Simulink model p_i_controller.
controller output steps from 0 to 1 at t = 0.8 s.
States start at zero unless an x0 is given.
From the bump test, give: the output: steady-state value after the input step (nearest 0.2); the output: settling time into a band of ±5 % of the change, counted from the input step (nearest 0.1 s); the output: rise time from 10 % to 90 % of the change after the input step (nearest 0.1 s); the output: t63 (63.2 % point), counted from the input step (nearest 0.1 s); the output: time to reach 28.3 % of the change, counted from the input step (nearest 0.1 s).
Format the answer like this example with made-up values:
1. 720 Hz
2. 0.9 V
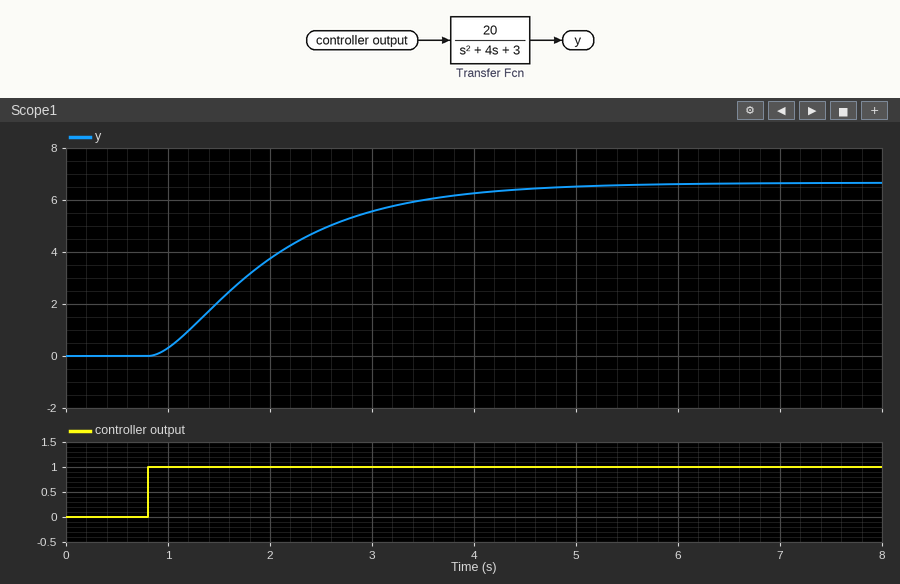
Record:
1. 6.6
2. 3.4 s
3. 2.4 s
4. 1.4 s
5. 0.6 s
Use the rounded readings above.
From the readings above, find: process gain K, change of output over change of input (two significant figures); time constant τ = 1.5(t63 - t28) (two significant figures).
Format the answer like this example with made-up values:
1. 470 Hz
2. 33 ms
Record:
1. 6.6
2. 1.2 s
